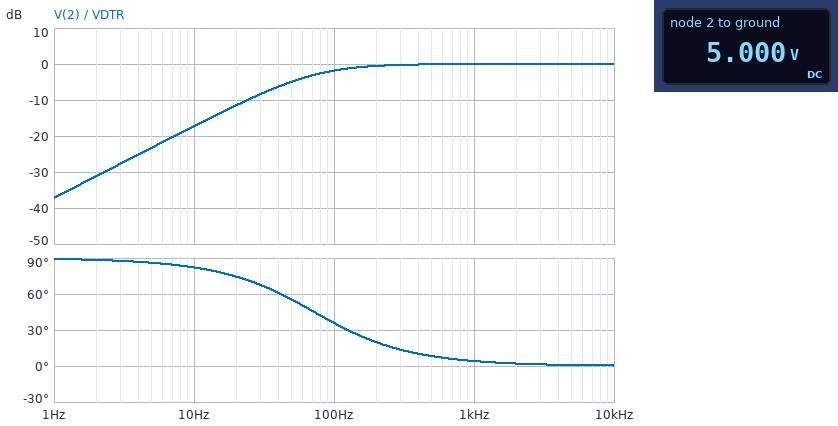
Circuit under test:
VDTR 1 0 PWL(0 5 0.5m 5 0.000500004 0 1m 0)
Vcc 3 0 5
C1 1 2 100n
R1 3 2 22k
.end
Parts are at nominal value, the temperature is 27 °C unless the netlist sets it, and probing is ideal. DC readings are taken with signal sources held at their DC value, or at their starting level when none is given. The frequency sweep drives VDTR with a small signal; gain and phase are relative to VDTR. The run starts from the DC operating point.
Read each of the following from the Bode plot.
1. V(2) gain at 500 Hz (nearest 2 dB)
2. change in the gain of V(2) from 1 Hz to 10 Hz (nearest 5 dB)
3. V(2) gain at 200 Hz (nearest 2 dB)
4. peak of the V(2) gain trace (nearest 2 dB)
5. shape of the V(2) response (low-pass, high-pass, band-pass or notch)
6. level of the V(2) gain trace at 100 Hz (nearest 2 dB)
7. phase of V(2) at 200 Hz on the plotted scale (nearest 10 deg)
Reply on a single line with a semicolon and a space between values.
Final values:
0 dB; 20 dB; 0 dB; 0 dB; high-pass; -2 dB; 20 deg
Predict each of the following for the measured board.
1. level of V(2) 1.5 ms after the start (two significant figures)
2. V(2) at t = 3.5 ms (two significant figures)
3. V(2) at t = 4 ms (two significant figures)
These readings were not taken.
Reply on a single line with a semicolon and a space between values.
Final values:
1.8 V; 3.7 V; 4.0 V
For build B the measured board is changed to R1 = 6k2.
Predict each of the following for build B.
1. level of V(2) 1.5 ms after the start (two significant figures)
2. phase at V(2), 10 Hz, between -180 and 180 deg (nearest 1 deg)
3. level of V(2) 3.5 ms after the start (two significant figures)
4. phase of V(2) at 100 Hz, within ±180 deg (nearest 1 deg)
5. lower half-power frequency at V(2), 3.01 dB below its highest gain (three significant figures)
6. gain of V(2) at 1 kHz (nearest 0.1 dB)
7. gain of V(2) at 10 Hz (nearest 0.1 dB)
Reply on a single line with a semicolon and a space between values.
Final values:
4.0 V; 88 deg; 5.0 V; 69 deg; 257 Hz; -0.3 dB; -28.2 dB
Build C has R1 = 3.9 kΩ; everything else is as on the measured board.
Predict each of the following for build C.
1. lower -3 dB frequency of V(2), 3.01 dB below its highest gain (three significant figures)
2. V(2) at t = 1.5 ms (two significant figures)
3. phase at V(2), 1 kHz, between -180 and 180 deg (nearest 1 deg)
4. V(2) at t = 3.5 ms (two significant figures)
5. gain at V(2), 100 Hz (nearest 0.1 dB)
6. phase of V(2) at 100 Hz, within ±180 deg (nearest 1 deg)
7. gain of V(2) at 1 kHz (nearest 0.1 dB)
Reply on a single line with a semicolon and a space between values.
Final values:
408 Hz; 4.6 V; 22 deg; 5.0 V; -12.5 dB; 76 deg; -0.7 dB
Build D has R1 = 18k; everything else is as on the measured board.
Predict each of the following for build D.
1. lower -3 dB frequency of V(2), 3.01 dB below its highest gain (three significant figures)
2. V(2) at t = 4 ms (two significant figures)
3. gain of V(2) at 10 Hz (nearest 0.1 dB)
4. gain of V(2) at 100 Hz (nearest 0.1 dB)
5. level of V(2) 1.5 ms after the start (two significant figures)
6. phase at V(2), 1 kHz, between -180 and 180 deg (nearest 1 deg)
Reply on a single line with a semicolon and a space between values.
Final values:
88.4 Hz; 4.3 V; -19.0 dB; -2.5 dB; 2.1 V; 5 deg
